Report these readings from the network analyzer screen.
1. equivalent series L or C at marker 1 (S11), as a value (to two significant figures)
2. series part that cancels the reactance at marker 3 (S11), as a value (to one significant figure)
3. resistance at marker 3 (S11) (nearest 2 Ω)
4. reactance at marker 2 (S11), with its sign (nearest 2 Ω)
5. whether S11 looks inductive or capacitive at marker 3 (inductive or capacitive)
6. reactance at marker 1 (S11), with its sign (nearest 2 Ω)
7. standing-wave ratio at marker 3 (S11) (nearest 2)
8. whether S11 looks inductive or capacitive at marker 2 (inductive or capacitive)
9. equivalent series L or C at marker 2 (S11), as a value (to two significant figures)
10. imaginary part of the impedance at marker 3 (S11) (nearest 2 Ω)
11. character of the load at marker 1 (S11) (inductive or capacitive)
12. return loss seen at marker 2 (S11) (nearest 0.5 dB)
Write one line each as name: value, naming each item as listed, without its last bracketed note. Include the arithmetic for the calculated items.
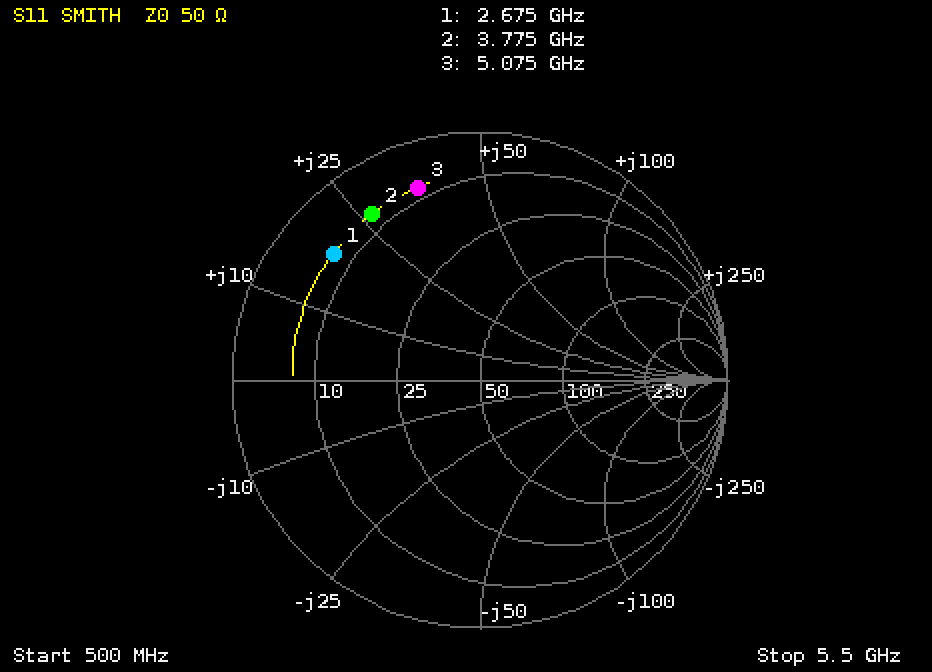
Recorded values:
equivalent series L or C at marker 1 (S11), as a value: L = 18 Ω/(2π × 2.675 GHz) ≈ 1.1 nH
series part that cancels the reactance at marker 3 (S11), as a value: C = 1/(2π × 5.075 GHz × 36 Ω) ≈ 871 fF, so 900 fF to one significant figure
resistance at marker 3 (S11): 8 Ω
reactance at marker 2 (S11), with its sign: +26 Ω
whether S11 looks inductive or capacitive at marker 3: inductive
reactance at marker 1 (S11), with its sign: +18 Ω
standing-wave ratio at marker 3 (S11): 10
whether S11 looks inductive or capacitive at marker 2: inductive
equivalent series L or C at marker 2 (S11), as a value: L = 26 Ω/(2π × 3.775 GHz) ≈ 1.1 nH
imaginary part of the impedance at marker 3 (S11): +36 Ω
character of the load at marker 1 (S11): inductive
return loss seen at marker 2 (S11): 2.0 dB
